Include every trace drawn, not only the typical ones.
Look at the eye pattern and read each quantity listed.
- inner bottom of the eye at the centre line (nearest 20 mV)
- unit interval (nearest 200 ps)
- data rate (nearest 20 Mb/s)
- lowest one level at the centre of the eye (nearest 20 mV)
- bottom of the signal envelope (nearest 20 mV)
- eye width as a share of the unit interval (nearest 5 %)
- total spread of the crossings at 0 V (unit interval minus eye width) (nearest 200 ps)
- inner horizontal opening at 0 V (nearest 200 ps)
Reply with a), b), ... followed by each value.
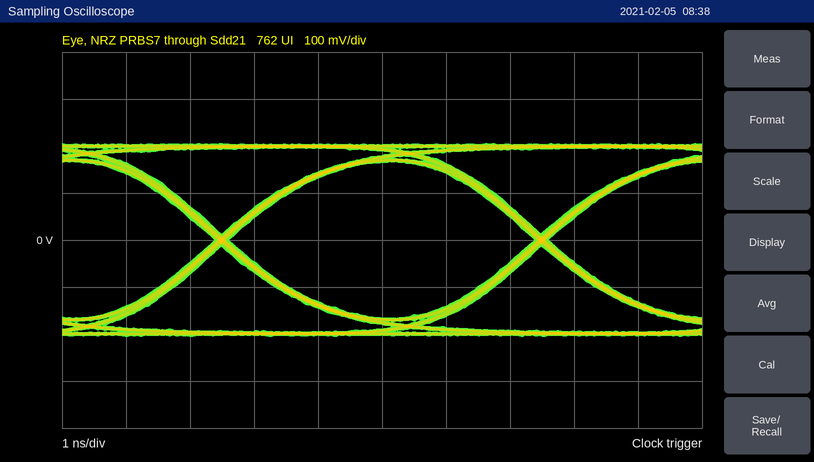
a) -160 mV
b) 5.0 ns
c) 200 Mb/s
d) 160 mV
e) -200 mV
f) 95 %
g) 200 ps
h) 4.8 ns
